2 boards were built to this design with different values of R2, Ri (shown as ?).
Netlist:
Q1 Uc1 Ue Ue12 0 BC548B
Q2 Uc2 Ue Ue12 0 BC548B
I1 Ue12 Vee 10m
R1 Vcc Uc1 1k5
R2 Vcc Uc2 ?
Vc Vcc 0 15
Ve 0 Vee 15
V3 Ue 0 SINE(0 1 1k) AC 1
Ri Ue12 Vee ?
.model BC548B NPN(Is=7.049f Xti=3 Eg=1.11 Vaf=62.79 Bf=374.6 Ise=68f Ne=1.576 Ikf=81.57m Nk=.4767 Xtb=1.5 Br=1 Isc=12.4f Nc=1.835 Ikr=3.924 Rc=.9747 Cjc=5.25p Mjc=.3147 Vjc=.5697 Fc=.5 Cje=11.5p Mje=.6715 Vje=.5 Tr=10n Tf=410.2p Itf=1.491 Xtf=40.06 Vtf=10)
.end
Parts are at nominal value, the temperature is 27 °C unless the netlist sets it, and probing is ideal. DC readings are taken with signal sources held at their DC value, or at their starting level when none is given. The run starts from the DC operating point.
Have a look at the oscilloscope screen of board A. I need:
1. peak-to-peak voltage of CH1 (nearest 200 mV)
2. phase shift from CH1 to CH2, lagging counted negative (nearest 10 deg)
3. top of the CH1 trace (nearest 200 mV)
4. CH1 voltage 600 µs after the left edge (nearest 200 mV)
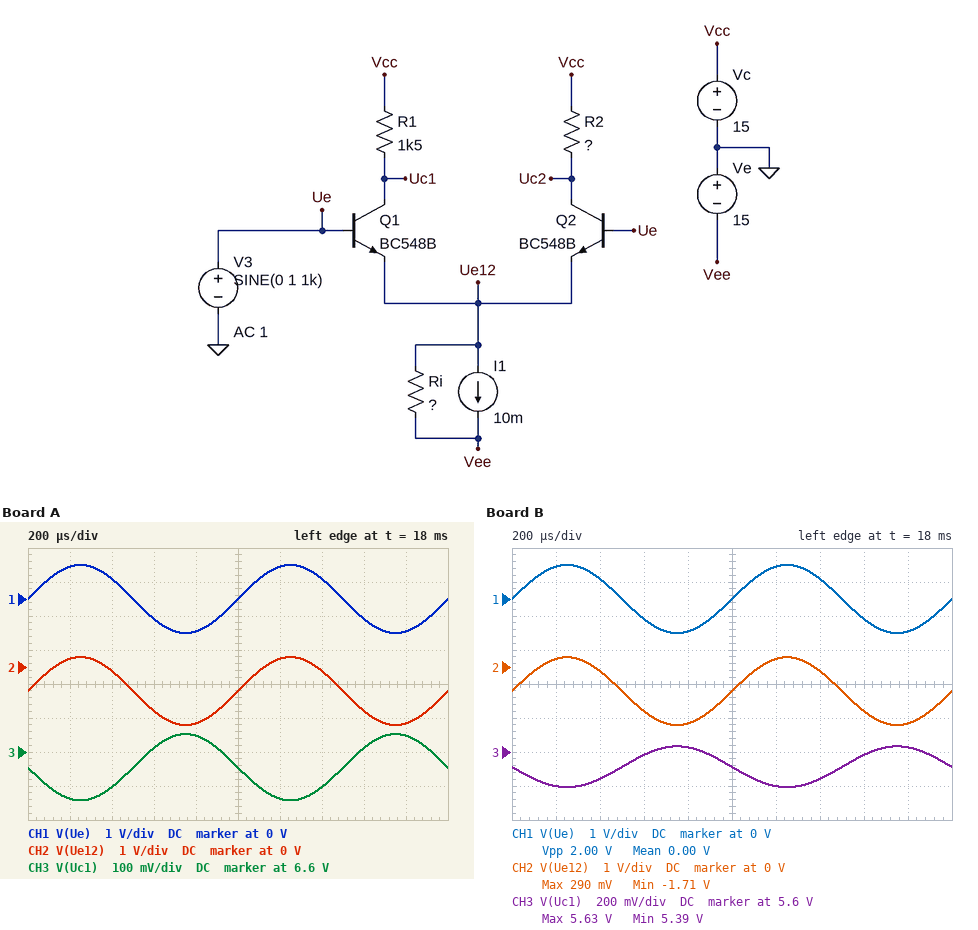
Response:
2.0 V
0 deg
1.0 V
-600 mV
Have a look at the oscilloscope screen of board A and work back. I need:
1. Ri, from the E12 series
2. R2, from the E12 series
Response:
68 kΩ
3.9 kΩ
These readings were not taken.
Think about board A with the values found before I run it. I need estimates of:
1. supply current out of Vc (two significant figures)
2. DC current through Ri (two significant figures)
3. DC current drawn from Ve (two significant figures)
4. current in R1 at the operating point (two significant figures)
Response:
9.6 mA
210 µA
10 mA
5.6 mA
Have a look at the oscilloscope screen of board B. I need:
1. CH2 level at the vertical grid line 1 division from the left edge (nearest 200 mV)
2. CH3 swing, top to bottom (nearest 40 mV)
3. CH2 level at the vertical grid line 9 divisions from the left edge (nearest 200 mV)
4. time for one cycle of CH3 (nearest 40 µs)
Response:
200 mV
240 mV
-1.6 V
1.00 ms
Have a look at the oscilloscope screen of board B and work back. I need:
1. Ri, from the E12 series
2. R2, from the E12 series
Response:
15 kΩ
4.7 kΩ
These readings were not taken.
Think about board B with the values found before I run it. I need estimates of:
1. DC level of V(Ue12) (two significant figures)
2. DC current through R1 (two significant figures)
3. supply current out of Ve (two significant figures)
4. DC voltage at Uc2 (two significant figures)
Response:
-710 mV
6.3 mA
11 mA
-670 mV
